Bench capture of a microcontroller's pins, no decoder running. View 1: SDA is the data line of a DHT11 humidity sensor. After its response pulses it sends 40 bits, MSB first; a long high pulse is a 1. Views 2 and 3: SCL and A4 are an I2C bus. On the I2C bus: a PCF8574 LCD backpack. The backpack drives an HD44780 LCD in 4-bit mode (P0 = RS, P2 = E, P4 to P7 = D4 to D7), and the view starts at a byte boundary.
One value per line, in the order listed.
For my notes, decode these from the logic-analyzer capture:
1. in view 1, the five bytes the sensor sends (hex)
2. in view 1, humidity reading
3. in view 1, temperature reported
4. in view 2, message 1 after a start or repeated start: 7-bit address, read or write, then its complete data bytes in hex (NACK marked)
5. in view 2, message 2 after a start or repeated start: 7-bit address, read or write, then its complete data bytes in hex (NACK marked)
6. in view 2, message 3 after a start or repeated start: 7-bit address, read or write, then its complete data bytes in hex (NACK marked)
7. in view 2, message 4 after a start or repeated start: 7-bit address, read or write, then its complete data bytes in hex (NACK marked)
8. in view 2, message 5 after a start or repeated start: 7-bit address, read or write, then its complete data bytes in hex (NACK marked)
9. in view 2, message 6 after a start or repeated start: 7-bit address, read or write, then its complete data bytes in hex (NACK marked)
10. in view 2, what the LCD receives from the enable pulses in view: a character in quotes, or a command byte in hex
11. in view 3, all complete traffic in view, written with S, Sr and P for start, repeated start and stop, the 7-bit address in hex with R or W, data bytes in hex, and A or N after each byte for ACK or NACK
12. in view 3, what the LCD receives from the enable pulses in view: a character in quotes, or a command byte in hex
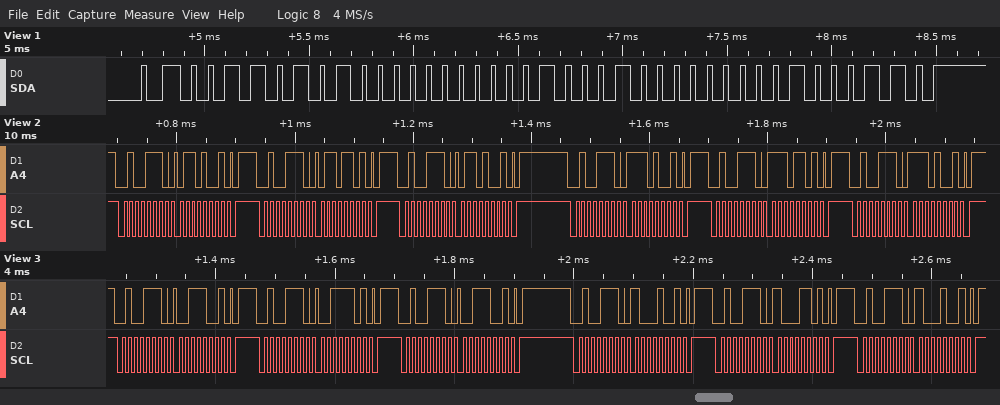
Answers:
35 00 11 00 46
53 %
17.0 °C
0x27 write: 69
0x27 write: 6D
0x27 write: 69
0x27 write: E9
0x27 write: ED
0x27 write: E9
'n'
S 27W A 39 A P S 27W A 3D A P S 27W A 39 A P S 27W A 89 A P S 27W A 8D A P S 27W A 89 A P
'8'
